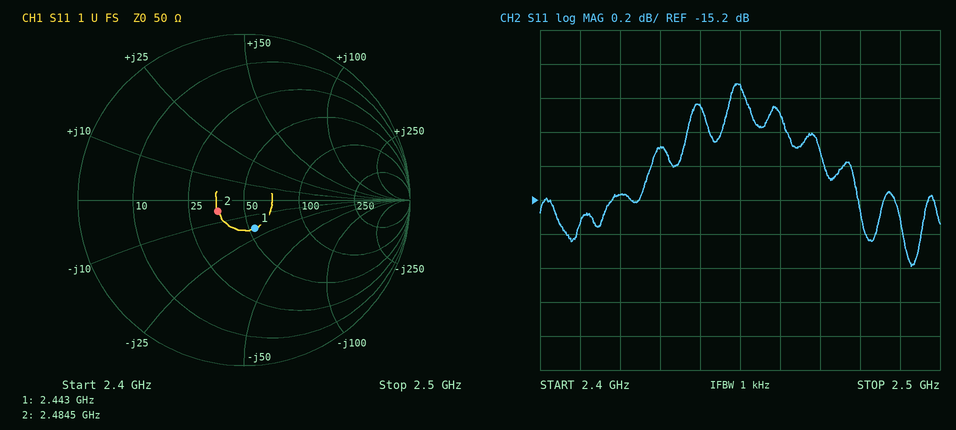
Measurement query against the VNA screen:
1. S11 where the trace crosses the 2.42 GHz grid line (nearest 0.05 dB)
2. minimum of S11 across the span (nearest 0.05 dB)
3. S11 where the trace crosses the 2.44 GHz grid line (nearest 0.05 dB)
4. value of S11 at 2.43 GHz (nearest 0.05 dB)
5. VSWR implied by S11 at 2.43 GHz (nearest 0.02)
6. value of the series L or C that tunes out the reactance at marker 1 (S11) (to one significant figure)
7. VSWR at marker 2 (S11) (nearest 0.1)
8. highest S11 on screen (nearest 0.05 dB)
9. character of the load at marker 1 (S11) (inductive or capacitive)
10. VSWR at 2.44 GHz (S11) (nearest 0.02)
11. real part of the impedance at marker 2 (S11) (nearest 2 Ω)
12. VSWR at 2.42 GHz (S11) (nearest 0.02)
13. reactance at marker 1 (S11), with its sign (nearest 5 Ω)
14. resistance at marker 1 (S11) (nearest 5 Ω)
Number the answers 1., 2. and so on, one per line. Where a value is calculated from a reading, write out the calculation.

1. -15.15 dB
2. -15.60 dB
3. -14.65 dB
4. -14.90 dB
5. |Γ| = 10^(-14.9/20) = 0.1799; VSWR = (1 + 0.1799)/(1 − 0.1799) ≈ 1.44
6. L = 20 Ω/(2π × 2.443 GHz) ≈ 1 nH
7. 1.4
8. -14.50 dB
9. capacitive
10. |Γ| = 10^(-14.65/20) = 0.1851; VSWR = (1 + 0.1851)/(1 − 0.1851) ≈ 1.45, so 1.46 to the nearest 0.02
11. 36 Ω
12. |Γ| = 10^(-15.15/20) = 0.1748; VSWR = (1 + 0.1748)/(1 − 0.1748) ≈ 1.42
13. -20 Ω
14. 55 Ω
